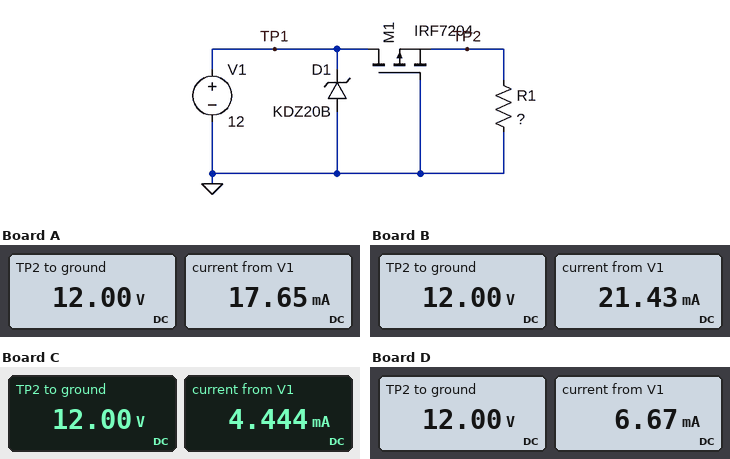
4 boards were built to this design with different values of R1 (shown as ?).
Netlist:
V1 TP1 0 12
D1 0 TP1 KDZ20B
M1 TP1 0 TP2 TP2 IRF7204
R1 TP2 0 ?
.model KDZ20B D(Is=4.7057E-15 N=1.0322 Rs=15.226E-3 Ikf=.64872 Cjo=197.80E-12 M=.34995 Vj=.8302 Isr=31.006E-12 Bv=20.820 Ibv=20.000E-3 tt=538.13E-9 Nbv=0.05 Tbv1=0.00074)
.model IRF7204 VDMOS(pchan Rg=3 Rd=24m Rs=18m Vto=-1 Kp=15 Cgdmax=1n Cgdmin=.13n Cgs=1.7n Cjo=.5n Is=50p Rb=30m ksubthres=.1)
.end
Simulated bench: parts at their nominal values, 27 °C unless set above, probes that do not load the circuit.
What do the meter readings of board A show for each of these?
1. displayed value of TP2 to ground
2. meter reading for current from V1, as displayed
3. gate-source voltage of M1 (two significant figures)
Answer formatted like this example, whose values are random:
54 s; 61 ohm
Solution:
12.00 V; 17.65 mA; -12 V
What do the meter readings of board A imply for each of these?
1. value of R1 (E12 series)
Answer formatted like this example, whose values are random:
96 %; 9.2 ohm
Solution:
680 Ω
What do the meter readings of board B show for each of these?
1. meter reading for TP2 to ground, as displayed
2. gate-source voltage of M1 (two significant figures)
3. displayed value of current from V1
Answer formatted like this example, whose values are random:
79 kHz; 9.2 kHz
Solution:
12.00 V; -12 V; 21.43 mA
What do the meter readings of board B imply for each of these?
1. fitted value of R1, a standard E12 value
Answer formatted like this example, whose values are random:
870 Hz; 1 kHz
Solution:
560 Ω
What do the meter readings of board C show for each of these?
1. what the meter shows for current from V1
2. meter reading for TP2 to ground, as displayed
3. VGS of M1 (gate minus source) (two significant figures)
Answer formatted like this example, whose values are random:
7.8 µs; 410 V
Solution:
4.444 mA; 12.00 V; -12 V
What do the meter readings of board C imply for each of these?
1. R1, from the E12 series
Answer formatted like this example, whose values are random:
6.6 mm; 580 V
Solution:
2.7 kΩ
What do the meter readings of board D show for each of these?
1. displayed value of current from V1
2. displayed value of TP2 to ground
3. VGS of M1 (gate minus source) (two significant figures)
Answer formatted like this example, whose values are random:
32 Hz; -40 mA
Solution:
6.67 mA; 12.00 V; -12 V
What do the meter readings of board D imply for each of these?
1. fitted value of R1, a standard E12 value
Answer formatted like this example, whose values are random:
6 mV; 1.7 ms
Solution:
1.8 kΩ
